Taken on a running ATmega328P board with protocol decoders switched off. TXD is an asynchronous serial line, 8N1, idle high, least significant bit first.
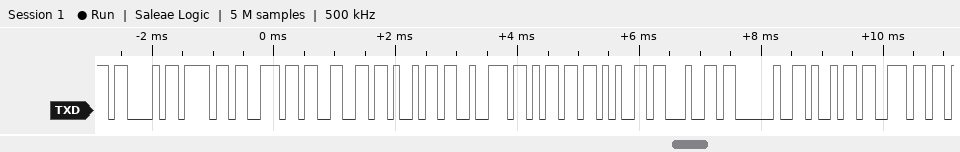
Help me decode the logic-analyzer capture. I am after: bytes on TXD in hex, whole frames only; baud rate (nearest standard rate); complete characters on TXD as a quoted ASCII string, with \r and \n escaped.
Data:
43 6F 6E 66 69 72 6D 65 64 20 69 6E
9600 baud
"Confirmed in"
